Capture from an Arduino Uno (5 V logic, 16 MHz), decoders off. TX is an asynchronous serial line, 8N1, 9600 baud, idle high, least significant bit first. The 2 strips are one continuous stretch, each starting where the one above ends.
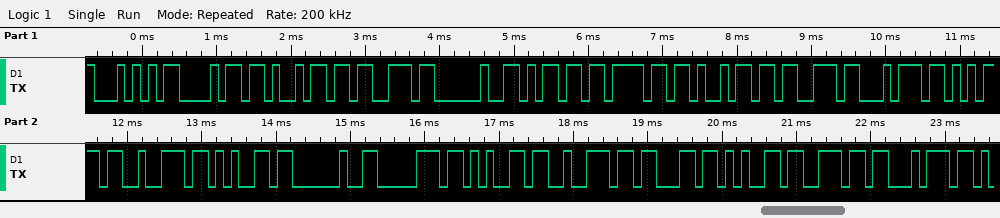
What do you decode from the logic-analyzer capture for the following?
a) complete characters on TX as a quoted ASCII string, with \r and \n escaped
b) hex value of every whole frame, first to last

"This moisture percent"
54 68 69 73 20 6D 6F 69 73 74 75 72 65 20 70 65 72 63 65 6E 74
